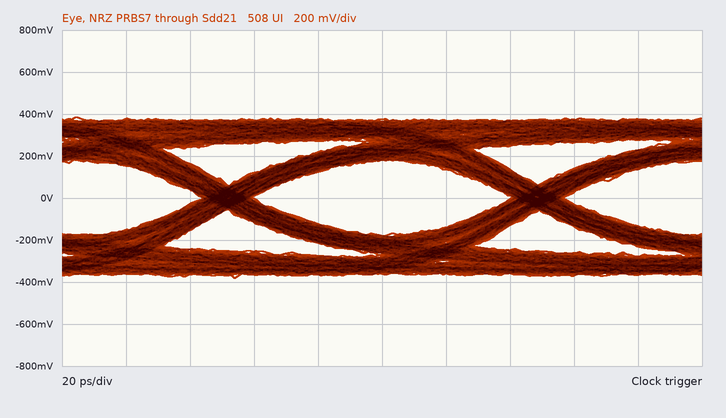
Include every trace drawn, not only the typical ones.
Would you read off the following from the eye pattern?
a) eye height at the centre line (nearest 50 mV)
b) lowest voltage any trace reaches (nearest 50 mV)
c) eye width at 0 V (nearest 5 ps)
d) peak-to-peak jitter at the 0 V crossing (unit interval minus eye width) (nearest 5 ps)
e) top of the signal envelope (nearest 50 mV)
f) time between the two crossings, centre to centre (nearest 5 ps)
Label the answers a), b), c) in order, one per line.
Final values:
a) 350 mV
b) -400 mV
c) 80 ps
d) 15 ps
e) 400 mV
f) 95 ps
